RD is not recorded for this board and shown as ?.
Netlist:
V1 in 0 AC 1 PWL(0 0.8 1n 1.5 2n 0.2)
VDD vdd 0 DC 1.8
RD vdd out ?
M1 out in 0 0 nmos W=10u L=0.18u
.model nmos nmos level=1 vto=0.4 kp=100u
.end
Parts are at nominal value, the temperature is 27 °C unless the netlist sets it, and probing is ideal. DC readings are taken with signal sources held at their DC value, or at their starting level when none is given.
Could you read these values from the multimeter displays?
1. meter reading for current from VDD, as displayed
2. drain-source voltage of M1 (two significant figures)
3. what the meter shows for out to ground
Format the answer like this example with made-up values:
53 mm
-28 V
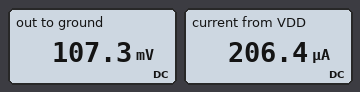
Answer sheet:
206.4 µA
110 mV
107.3 mV
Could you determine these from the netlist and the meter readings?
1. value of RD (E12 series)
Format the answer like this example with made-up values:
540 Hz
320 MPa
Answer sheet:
8.2 kΩ
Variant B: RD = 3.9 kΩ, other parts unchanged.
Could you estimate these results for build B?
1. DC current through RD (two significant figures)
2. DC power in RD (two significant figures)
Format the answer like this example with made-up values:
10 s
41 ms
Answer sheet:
390 µA
600 µW
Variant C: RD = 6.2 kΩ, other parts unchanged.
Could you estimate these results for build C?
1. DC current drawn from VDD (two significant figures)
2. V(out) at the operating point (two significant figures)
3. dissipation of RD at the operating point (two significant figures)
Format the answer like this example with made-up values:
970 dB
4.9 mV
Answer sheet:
270 µA
150 mV
440 µW
